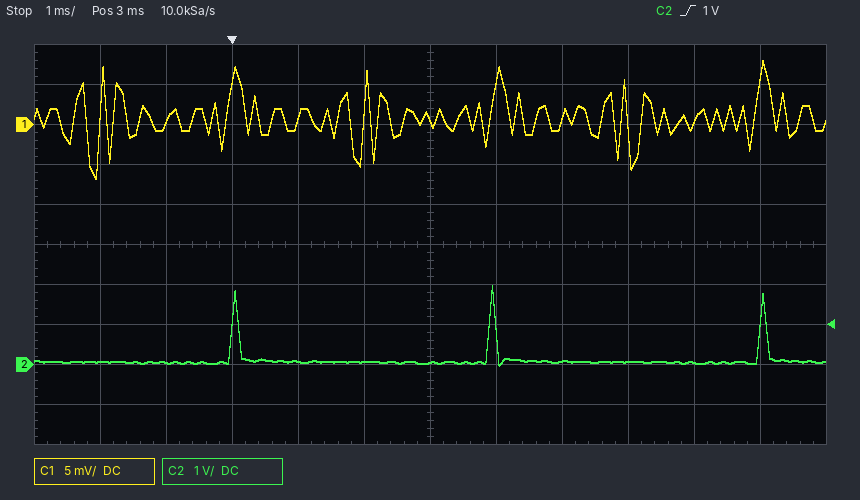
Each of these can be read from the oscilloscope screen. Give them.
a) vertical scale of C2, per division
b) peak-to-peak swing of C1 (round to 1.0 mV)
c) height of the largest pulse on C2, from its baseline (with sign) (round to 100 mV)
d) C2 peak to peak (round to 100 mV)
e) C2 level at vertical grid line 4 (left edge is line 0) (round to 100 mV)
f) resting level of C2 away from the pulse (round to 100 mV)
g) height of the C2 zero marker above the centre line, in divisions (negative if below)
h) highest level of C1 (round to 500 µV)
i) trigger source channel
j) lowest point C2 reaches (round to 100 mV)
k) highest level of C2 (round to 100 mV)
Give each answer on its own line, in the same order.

1 V
15.0 mV
+1.9 V
2.0 V
100 mV
100 mV
-3.0 div
8.0 mV
C2
0.0 V
2.0 V
